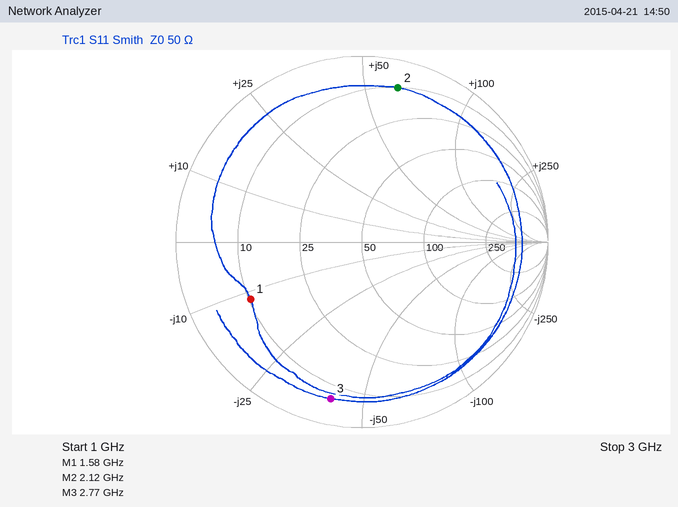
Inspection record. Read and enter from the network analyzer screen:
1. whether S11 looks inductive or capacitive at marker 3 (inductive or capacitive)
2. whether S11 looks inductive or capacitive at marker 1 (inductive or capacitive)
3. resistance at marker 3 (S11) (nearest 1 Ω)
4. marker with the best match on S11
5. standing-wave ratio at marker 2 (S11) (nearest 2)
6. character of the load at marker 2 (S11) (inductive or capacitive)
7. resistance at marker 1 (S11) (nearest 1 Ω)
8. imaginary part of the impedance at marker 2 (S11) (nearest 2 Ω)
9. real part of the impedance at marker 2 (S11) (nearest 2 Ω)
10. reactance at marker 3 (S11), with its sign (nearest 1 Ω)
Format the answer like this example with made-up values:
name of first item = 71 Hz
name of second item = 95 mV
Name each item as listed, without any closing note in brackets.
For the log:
whether S11 looks inductive or capacitive at marker 3 = capacitive
whether S11 looks inductive or capacitive at marker 1 = capacitive
resistance at marker 3 (S11) = 6 Ω
marker with the best match on S11 = marker 1
standing-wave ratio at marker 2 (S11) = 12
character of the load at marker 2 (S11) = inductive
resistance at marker 1 (S11) = 10 Ω
imaginary part of the impedance at marker 2 (S11) = +62 Ω
real part of the impedance at marker 2 (S11) = 10 Ω
reactance at marker 3 (S11), with its sign = -41 Ω
